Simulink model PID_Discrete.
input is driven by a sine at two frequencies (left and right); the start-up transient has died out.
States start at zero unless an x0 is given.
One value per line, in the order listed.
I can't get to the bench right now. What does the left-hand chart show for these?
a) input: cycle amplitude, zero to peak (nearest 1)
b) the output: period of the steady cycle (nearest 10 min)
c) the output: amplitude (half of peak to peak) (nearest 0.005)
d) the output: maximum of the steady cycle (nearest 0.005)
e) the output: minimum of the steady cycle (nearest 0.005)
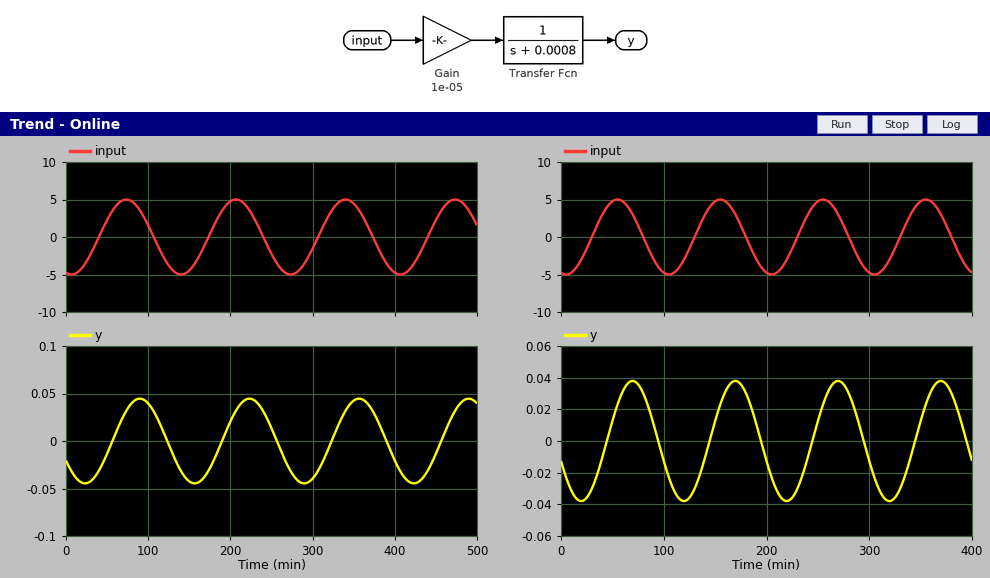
5
130 min
0.045
0.045
-0.045
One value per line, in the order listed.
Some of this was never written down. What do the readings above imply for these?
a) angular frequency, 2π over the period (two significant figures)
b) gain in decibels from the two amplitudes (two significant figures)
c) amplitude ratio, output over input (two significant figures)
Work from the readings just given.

0.048 rad/min
-41 dB
0.0090
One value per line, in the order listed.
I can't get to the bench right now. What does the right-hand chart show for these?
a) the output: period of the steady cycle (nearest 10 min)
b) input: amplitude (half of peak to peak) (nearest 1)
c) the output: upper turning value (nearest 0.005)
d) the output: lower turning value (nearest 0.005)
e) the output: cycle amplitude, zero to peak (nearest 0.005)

100 min
5
0.040
-0.040
0.040
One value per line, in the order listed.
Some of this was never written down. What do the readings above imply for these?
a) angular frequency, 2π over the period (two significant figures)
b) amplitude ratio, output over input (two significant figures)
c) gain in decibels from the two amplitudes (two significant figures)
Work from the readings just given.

0.063 rad/min
0.0080
-42 dB
